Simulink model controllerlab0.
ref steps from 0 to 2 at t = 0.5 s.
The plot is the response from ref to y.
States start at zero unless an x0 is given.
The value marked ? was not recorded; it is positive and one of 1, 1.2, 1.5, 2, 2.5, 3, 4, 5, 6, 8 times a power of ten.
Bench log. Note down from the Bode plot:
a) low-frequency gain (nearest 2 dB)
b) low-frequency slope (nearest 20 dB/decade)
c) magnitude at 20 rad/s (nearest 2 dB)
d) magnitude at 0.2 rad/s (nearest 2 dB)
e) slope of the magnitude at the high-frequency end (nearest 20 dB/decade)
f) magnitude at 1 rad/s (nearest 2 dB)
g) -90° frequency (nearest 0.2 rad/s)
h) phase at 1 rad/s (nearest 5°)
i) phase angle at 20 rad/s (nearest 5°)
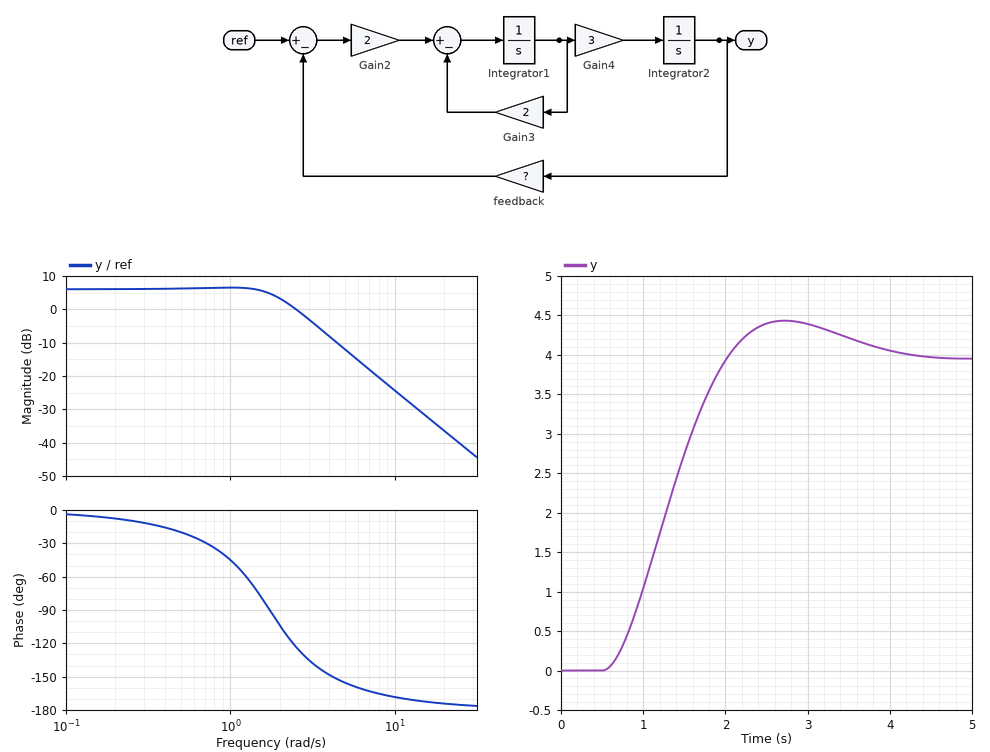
6 dB
0 dB/decade
-36 dB
6 dB
-40 dB/decade
6 dB
1.8 rad/s
-45°
-175°
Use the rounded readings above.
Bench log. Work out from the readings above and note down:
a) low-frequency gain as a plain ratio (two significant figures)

2.0
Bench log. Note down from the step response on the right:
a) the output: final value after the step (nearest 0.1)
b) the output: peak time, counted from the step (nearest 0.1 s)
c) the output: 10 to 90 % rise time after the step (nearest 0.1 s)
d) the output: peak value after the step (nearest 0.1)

4.0
2.2 s
1.0 s
4.4
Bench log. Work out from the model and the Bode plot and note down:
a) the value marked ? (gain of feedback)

0.5
